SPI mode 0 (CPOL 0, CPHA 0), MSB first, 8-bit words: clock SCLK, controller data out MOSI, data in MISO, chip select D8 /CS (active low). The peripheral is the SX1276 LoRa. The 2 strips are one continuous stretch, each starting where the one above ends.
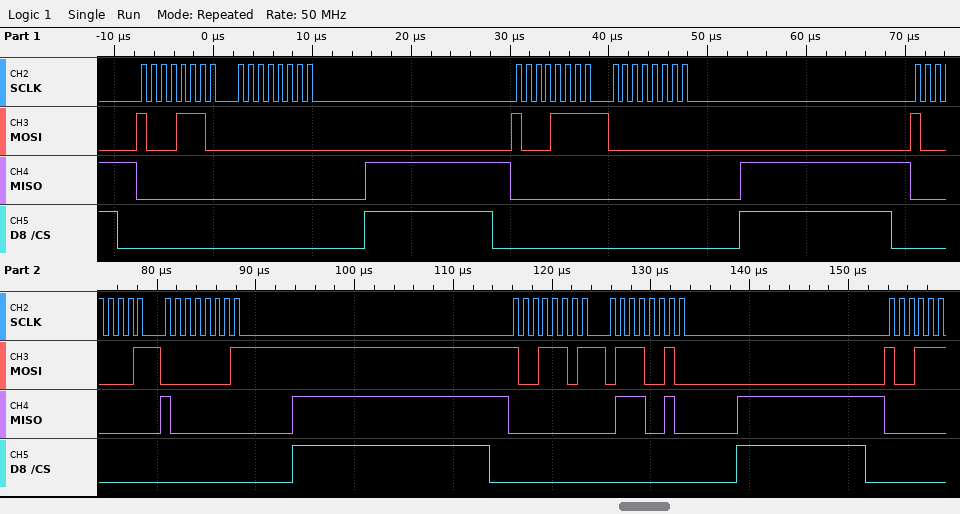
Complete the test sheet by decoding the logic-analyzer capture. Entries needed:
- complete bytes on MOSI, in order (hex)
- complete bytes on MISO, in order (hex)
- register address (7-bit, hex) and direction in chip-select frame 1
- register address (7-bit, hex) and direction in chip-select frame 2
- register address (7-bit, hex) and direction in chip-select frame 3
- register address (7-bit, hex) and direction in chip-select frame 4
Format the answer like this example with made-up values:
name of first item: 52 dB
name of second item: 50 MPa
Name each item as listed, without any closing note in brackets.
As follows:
complete bytes on MOSI, in order: 8E 00 8F 00 81 01 9D 72
complete bytes on MISO, in order: 00 00 00 00 00 80 00 72
register address (7-bit, hex) and direction in chip-select frame 1: 0x0E write
register address (7-bit, hex) and direction in chip-select frame 2: 0x0F write
register address (7-bit, hex) and direction in chip-select frame 3: 0x01 write
register address (7-bit, hex) and direction in chip-select frame 4: 0x1D write
